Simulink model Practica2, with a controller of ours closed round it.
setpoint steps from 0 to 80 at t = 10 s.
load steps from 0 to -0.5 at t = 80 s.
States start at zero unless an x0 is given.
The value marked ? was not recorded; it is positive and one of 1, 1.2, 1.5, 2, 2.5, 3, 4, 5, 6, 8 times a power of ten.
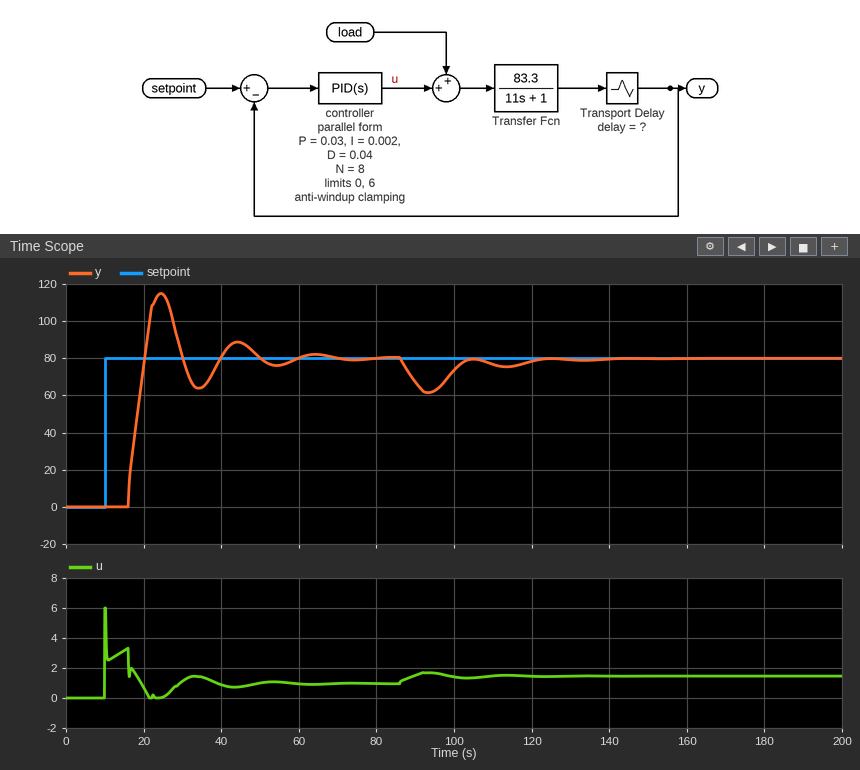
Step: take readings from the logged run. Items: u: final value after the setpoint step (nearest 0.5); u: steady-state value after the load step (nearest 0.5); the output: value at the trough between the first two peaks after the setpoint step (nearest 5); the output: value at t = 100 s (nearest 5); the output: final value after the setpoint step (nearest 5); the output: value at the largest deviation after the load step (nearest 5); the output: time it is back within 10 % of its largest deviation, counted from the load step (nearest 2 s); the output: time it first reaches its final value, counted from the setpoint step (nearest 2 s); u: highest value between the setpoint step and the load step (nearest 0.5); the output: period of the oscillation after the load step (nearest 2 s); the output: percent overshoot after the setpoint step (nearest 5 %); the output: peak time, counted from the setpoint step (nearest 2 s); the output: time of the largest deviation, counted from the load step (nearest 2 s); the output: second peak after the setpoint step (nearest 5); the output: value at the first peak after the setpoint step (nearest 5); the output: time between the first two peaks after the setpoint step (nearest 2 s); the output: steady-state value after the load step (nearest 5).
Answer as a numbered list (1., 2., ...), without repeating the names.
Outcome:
1. 1.0
2. 1.5
3. 65
4. 75
5. 80
6. 60
7. 40 s
8. 10 s
9. 6.0
10. 20 s
11. 45 %
12. 14 s
13. 14 s
14. 90
15. 115
16. 20 s
17. 80
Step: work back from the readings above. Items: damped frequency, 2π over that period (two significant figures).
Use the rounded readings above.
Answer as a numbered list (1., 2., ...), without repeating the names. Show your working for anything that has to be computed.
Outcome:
1. 2π / 20 = 0.31 rad/s
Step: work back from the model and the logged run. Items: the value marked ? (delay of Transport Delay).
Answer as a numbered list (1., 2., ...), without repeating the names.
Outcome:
1. 6
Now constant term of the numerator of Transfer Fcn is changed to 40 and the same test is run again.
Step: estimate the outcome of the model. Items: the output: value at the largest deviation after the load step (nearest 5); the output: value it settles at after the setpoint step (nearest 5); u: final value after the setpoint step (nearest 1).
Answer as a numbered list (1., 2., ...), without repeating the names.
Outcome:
1. 70
2. 80
3. 2
